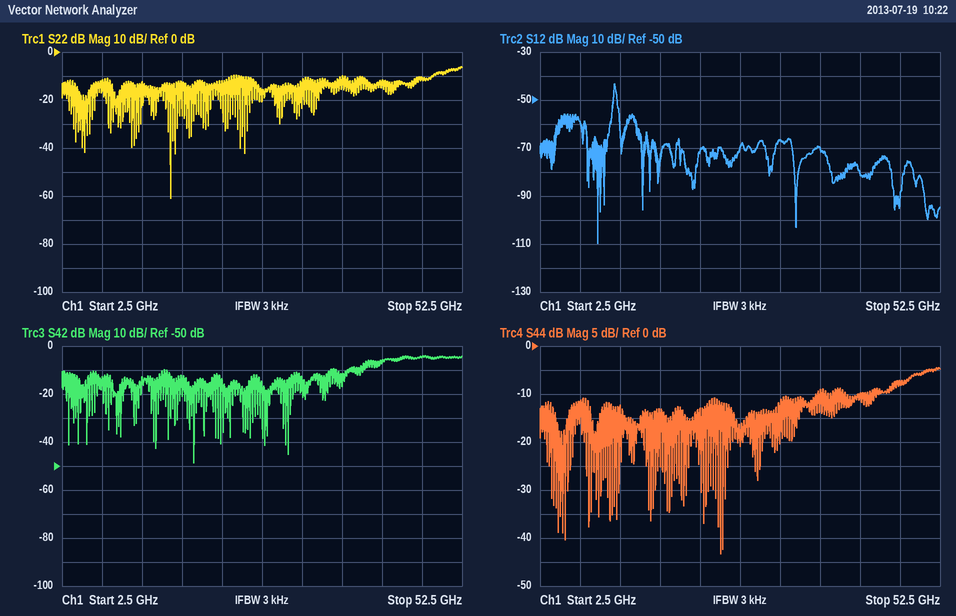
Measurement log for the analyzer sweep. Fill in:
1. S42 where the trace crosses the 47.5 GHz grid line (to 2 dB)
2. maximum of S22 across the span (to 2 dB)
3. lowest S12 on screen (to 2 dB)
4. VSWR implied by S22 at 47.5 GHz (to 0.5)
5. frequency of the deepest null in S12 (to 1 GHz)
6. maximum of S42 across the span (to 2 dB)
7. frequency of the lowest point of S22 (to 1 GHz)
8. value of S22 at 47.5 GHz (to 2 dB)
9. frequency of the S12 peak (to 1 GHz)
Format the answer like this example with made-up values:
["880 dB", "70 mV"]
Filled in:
["-4 dB", "-6 dB", "-110 dB", "2.0", "10 GHz", "-4 dB", "16 GHz", "-10 dB", "12 GHz"]
